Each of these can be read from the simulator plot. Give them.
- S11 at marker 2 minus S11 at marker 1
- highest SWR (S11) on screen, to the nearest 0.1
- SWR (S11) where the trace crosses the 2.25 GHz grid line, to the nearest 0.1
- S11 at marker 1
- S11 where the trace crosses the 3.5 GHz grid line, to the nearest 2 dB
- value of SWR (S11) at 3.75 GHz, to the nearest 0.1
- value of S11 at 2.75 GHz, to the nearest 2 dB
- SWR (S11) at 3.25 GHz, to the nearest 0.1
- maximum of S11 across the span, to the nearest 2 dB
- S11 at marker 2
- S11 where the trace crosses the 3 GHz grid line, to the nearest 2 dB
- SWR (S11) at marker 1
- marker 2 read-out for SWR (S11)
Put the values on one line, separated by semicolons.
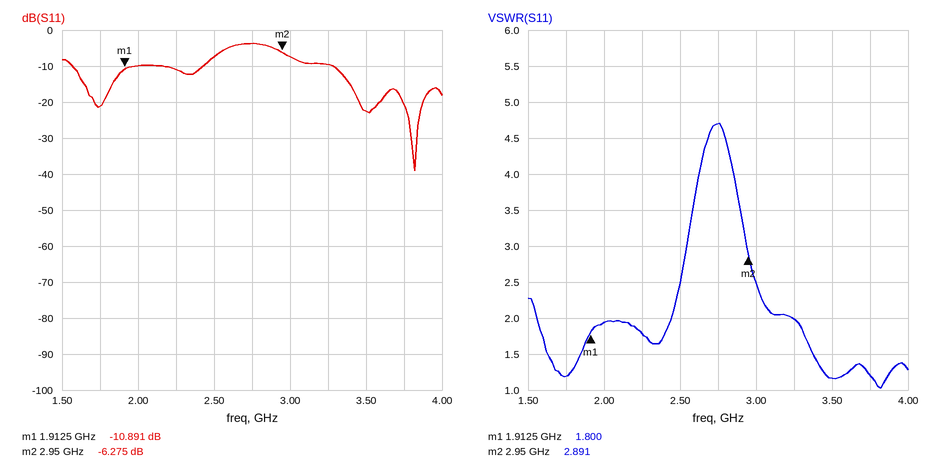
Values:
4.616 dB; 4.7; 1.8; -10.891 dB; -22 dB; 1.2; -4 dB; 2.0; -4 dB; -6.275 dB; -8 dB; 1.800; 2.891
